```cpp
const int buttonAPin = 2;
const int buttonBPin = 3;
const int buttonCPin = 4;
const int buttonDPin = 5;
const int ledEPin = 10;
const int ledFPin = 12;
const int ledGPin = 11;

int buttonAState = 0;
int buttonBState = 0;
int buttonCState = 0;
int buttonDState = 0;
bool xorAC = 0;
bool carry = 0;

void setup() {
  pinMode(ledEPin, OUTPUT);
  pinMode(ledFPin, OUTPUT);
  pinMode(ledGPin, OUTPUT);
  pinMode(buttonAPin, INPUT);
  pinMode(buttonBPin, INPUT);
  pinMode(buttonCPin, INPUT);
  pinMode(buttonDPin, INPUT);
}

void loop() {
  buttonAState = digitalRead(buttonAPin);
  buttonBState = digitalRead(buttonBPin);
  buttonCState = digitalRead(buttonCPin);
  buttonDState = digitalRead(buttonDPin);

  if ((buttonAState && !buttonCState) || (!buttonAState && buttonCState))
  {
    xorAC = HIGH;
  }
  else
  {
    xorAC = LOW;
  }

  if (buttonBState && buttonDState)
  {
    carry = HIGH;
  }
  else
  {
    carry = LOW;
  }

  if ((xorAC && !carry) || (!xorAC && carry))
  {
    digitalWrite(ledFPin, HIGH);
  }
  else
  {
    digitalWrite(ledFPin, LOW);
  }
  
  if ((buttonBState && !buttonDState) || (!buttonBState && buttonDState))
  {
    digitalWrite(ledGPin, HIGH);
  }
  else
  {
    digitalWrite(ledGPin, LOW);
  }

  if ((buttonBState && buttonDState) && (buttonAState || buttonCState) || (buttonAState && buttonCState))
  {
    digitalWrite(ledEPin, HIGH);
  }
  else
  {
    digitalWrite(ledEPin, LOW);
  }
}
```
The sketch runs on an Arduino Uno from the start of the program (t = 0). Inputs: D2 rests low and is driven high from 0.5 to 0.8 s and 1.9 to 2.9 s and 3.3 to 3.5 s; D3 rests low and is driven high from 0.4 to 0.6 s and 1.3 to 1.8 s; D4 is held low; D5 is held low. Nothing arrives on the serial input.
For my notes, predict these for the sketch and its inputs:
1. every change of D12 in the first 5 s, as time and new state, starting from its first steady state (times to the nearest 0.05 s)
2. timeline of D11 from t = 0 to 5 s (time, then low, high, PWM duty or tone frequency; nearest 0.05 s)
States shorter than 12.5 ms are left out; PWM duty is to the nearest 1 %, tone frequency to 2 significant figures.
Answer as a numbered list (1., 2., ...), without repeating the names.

1. 0 s low; 0.5 s high; 0.8 s low; 1.9 s high; 2.9 s low; 3.3 s high; 3.5 s low
2. 0 s low; 0.4 s high; 0.6 s low; 1.3 s high; 1.8 s low
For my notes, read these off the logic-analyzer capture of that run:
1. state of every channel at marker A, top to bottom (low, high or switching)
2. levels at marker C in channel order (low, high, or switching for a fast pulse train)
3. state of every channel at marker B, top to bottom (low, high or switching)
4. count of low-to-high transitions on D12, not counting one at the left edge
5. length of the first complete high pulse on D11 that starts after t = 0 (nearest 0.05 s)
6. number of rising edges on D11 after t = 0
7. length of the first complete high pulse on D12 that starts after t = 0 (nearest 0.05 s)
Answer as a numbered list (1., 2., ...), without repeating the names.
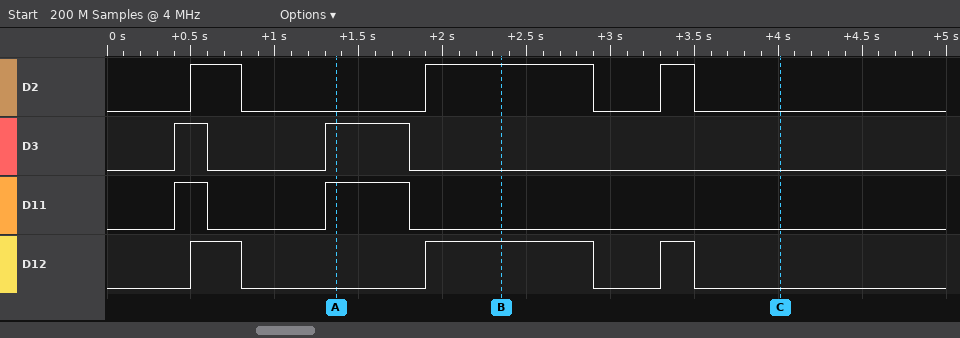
1. D2 low, D3 high, D11 high, D12 low
2. D2 low, D3 low, D11 low, D12 low
3. D2 high, D3 low, D11 low, D12 high
4. 3
5. 0.20 s
6. 2
7. 0.30 s
